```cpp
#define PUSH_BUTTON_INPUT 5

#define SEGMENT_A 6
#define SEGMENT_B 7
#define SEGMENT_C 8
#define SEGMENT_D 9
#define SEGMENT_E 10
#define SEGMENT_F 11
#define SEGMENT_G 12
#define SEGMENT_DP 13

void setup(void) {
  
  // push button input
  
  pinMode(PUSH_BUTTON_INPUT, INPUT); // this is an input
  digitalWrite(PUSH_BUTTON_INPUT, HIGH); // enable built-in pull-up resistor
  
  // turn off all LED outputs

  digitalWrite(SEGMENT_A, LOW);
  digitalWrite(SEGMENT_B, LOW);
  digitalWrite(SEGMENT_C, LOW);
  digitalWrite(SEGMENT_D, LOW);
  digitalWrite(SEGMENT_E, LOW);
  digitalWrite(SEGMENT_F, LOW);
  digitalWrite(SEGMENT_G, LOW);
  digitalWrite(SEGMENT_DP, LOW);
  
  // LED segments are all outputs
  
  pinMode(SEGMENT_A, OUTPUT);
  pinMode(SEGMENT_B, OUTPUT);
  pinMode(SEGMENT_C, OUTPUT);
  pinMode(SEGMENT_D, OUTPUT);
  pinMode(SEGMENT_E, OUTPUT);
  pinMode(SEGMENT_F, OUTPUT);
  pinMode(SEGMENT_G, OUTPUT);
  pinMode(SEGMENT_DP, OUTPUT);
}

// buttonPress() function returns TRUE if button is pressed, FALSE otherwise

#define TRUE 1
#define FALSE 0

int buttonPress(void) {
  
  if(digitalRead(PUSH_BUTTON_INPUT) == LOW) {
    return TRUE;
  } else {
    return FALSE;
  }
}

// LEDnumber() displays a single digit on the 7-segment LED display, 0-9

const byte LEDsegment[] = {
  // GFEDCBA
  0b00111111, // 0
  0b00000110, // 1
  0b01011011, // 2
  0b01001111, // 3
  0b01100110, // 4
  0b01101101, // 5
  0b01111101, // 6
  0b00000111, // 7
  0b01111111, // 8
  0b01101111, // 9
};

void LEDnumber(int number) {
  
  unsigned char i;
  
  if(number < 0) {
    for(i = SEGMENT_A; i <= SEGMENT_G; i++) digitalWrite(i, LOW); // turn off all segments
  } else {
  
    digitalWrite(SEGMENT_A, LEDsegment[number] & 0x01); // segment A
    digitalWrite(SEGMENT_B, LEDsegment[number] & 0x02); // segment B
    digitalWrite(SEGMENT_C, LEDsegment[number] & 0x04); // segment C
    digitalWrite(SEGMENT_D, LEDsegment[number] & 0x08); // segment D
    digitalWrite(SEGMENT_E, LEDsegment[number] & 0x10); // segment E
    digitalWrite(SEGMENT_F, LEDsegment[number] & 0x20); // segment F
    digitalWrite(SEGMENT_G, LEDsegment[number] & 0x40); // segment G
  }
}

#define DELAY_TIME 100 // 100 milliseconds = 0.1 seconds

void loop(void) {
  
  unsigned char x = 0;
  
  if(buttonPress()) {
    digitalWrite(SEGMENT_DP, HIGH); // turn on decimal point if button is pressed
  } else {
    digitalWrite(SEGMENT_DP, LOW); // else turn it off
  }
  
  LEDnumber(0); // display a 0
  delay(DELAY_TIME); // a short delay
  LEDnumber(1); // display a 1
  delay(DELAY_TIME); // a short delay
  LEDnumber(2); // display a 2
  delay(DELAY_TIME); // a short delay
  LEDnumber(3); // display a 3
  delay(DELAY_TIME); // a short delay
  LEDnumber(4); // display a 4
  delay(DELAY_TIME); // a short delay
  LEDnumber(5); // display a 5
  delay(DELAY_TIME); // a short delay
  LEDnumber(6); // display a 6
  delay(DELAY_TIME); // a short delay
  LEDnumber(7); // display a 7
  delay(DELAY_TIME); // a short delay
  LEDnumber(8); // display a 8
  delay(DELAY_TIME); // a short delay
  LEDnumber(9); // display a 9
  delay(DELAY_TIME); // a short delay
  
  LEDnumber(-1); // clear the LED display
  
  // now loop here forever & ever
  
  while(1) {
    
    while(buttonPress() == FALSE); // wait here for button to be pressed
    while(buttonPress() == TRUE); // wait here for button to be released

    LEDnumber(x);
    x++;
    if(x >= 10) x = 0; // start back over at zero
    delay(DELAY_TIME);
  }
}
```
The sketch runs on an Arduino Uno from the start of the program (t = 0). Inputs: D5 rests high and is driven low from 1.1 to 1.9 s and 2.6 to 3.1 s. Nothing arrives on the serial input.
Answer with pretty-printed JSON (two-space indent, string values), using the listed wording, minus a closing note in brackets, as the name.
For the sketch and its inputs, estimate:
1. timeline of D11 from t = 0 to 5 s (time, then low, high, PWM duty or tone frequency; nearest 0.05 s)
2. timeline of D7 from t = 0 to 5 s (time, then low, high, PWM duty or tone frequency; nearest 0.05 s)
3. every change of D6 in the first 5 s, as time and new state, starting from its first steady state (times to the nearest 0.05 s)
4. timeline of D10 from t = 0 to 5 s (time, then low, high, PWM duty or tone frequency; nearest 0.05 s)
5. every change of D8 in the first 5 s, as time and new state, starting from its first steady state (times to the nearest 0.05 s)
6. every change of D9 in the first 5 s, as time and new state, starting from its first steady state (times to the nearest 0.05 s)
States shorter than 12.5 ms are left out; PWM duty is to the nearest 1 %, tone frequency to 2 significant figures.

{
  "timeline of D11 from t = 0 to 5 s": "0 s high; 0.1 s low; 0.4 s high; 0.7 s low; 0.8 s high; 1 s low; 1.9 s high; 3.1 s low",
  "timeline of D7 from t = 0 to 5 s": "0 s high; 0.5 s low; 0.7 s high; 1 s low; 1.9 s high",
  "every change of D6 in the first 5 s, as time and new state, starting from its first steady state": "0 s high; 0.1 s low; 0.2 s high; 0.4 s low; 0.5 s high; 1 s low; 1.9 s high; 3.1 s low",
  "timeline of D10 from t = 0 to 5 s": "0 s high; 0.1 s low; 0.2 s high; 0.3 s low; 0.6 s high; 0.7 s low; 0.8 s high; 0.9 s low; 1.9 s high; 3.1 s low",
  "every change of D8 in the first 5 s, as time and new state, starting from its first steady state": "0 s high; 0.2 s low; 0.3 s high; 1 s low; 1.9 s high",
  "every change of D9 in the first 5 s, as time and new state, starting from its first steady state": "0 s high; 0.1 s low; 0.2 s high; 0.4 s low; 0.5 s high; 0.7 s low; 0.8 s high; 1 s low; 1.9 s high; 3.1 s low"
}
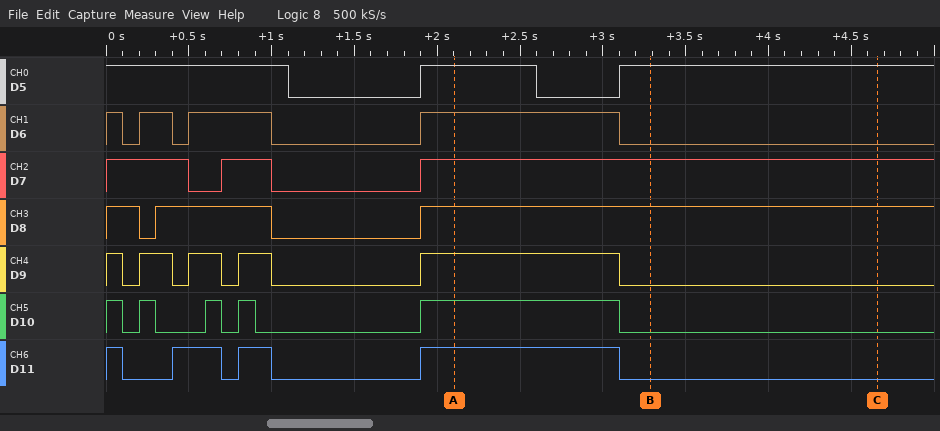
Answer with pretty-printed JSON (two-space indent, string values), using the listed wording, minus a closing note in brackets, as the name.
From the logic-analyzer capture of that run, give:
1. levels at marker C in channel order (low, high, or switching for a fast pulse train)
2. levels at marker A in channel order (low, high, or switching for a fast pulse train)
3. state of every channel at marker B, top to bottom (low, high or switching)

{
  "levels at marker C in channel order": "D5 high, D6 low, D7 high, D8 high, D9 low, D10 low, D11 low",
  "levels at marker A in channel order": "D5 high, D6 high, D7 high, D8 high, D9 high, D10 high, D11 high",
  "state of every channel at marker B, top to bottom": "D5 high, D6 low, D7 high, D8 high, D9 low, D10 low, D11 low"
}
